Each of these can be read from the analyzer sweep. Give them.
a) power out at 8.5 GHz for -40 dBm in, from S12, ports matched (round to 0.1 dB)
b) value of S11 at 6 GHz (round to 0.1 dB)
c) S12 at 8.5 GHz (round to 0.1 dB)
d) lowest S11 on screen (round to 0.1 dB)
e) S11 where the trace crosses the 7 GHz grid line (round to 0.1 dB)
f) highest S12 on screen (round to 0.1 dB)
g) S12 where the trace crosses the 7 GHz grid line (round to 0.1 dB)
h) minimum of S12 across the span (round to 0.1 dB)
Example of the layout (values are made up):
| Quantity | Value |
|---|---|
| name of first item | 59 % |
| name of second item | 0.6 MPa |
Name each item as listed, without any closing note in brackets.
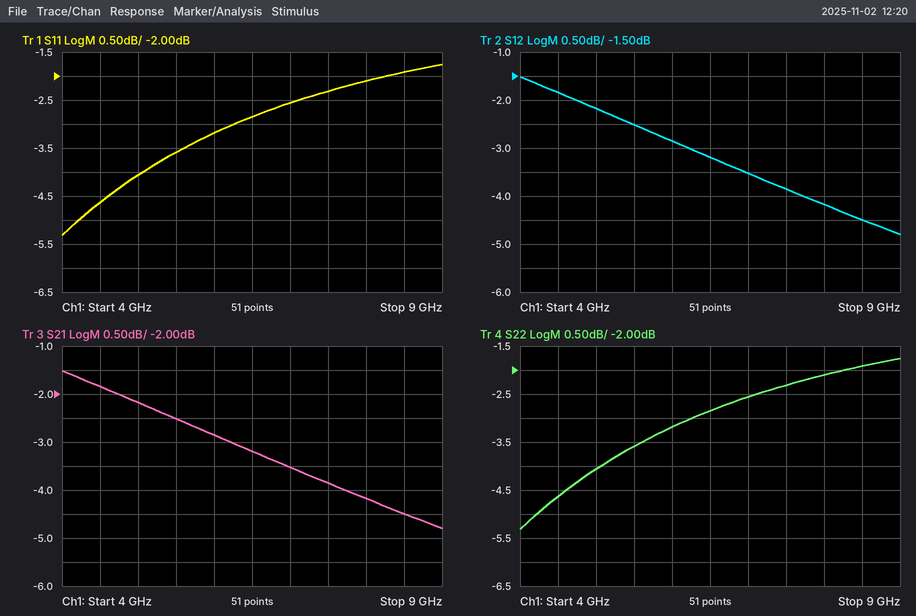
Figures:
| Quantity | Value |
|---|---|
| power out at 8.5 GHz for -40 dBm in, from S12, ports matched | -44.5 dBm |
| value of S11 at 6 GHz | -3.2 dB |
| S12 at 8.5 GHz | -4.5 dB |
| lowest S11 on screen | -5.3 dB |
| S11 where the trace crosses the 7 GHz grid line | -2.6 dB |
| highest S12 on screen | -1.5 dB |
| S12 where the trace crosses the 7 GHz grid line | -3.5 dB |
| minimum of S12 across the span | -4.8 dB |
